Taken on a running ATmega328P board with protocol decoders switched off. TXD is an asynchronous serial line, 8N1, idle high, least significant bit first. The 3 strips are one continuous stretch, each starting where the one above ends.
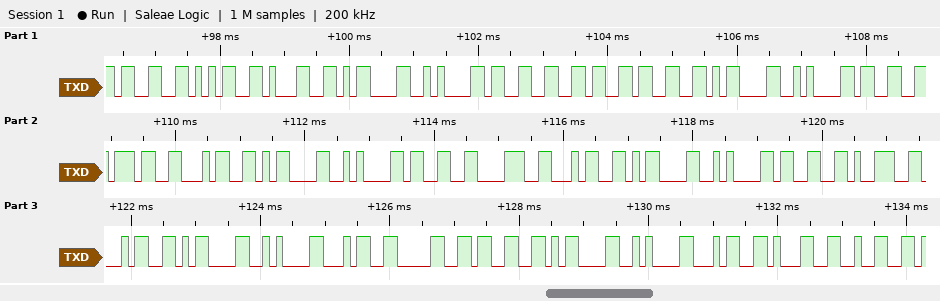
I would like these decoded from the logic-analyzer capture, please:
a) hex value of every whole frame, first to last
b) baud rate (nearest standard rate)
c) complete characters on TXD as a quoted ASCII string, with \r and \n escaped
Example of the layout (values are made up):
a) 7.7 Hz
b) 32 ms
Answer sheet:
a) 33 35 31 0D 0A 33 36 33 0D 0A 33 37 34 0D 0A 33 38 34 0D 0A 33 39 34 0D 0A 34 30 33 0D 0A 34 31 32
b) 9600 baud
c) "351\r\n363\r\n374\r\n384\r\n394\r\n403\r\n412"
